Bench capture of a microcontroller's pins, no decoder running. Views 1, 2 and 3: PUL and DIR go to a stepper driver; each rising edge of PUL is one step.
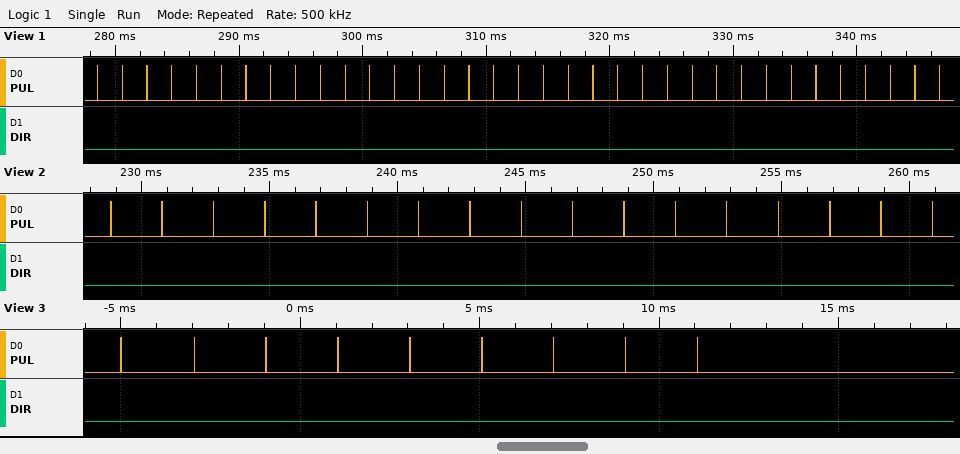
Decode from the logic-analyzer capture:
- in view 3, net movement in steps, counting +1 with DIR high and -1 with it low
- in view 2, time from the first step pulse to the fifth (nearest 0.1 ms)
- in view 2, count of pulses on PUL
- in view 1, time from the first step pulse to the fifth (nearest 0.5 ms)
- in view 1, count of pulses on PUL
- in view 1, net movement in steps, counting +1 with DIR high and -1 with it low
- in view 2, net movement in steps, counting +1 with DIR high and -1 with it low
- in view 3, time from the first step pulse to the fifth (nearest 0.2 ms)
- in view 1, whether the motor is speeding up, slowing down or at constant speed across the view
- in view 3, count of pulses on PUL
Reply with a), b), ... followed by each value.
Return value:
a) -9
b) 8.0 ms
c) 17
d) 8.0 ms
e) 35
f) -35
g) -17
h) 8.0 ms
i) constant speed
j) 9
